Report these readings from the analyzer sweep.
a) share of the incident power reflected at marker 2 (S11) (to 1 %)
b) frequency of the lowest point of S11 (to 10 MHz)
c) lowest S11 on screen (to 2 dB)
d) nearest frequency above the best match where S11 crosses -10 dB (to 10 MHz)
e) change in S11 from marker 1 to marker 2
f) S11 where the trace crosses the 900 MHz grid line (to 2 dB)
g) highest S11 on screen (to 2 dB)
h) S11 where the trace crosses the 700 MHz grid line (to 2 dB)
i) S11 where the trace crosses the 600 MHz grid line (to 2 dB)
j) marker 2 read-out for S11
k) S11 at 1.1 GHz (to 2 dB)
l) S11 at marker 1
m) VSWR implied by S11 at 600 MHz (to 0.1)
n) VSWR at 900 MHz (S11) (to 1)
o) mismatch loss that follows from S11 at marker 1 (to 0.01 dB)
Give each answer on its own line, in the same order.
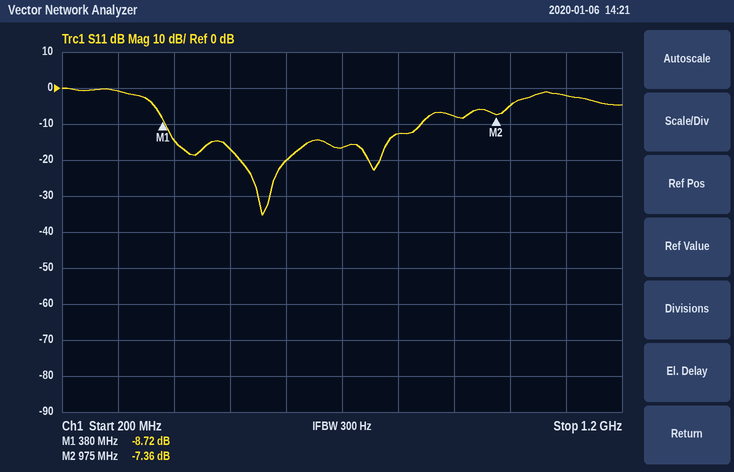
18 %
560 MHz
-36 dB
840 MHz
1.36 dB
-8 dB
0 dB
-16 dB
-20 dB
-7.36 dB
-2 dB
-8.72 dB
1.2
2
0.63 dB
